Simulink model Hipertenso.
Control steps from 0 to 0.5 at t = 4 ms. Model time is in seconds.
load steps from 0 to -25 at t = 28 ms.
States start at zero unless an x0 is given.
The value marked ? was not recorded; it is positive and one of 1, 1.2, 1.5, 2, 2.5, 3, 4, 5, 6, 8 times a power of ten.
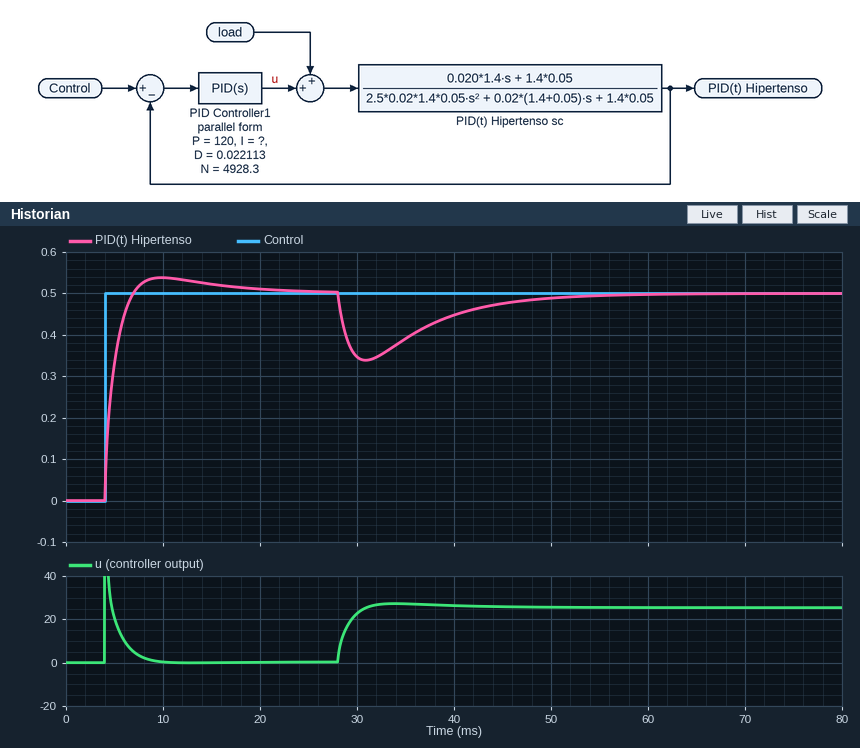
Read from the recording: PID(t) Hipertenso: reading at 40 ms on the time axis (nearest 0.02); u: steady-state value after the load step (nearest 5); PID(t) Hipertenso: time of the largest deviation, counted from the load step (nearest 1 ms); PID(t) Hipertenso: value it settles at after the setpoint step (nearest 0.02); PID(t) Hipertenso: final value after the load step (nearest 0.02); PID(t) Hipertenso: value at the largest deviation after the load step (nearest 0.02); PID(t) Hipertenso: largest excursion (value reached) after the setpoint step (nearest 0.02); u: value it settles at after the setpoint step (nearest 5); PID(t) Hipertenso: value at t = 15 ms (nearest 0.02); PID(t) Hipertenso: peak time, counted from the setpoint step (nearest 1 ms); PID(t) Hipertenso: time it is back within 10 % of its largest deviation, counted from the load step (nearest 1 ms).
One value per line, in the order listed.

0.44
25
3 ms
0.50
0.50
0.34
0.54
0
0.52
6 ms
20 ms
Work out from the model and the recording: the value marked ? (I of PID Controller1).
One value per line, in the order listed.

15000
